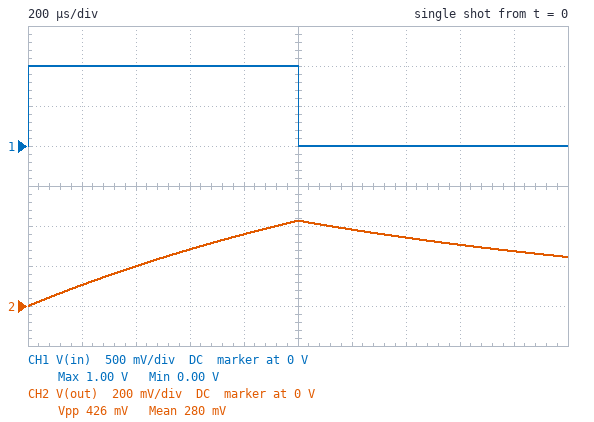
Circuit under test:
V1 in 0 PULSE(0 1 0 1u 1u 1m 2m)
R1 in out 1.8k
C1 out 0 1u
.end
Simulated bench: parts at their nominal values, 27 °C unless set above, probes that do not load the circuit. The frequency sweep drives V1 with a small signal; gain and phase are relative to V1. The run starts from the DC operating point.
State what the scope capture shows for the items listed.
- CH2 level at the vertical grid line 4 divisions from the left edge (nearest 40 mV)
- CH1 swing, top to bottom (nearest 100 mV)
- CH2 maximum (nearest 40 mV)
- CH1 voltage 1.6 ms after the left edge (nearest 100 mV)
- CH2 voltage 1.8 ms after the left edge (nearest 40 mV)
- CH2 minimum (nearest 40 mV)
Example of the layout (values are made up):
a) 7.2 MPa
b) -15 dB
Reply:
a) 360 mV
b) 1.0 V
c) 440 mV
d) 0 V
e) 280 mV
f) 0 V
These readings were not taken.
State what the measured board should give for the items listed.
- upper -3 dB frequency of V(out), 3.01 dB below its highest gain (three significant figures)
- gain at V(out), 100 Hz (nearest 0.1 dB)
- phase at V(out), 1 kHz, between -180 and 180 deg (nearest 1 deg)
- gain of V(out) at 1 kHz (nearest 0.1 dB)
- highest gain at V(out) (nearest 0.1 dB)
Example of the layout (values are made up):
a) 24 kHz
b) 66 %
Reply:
a) 88.4 Hz
b) -3.6 dB
c) -85 deg
d) -21.1 dB
e) 0 dB
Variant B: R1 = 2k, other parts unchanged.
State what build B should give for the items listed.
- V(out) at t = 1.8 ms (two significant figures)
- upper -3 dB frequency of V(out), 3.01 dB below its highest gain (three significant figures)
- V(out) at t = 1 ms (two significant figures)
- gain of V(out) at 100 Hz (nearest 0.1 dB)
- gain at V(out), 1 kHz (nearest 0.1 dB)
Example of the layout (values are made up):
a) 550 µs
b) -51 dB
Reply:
a) 260 mV
b) 79.6 Hz
c) 390 mV
d) -4.1 dB
e) -22.0 dB
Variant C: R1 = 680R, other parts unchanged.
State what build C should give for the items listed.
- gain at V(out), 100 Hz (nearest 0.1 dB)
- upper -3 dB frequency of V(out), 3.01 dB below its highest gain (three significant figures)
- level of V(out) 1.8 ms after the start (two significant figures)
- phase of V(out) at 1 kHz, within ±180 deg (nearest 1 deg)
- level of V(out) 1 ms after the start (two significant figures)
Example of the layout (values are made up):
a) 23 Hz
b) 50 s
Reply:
a) -0.7 dB
b) 234 Hz
c) 240 mV
d) -77 deg
e) 770 mV
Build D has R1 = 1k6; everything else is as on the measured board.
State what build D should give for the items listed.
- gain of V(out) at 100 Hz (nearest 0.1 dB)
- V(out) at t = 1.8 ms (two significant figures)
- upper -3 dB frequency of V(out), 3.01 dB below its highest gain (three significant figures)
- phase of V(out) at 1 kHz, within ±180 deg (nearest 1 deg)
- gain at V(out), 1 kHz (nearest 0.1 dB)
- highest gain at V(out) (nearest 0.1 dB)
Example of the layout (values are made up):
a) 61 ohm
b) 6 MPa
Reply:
a) -3.0 dB
b) 280 mV
c) 99.5 Hz
d) -84 deg
e) -20.1 dB
f) 0 dB
